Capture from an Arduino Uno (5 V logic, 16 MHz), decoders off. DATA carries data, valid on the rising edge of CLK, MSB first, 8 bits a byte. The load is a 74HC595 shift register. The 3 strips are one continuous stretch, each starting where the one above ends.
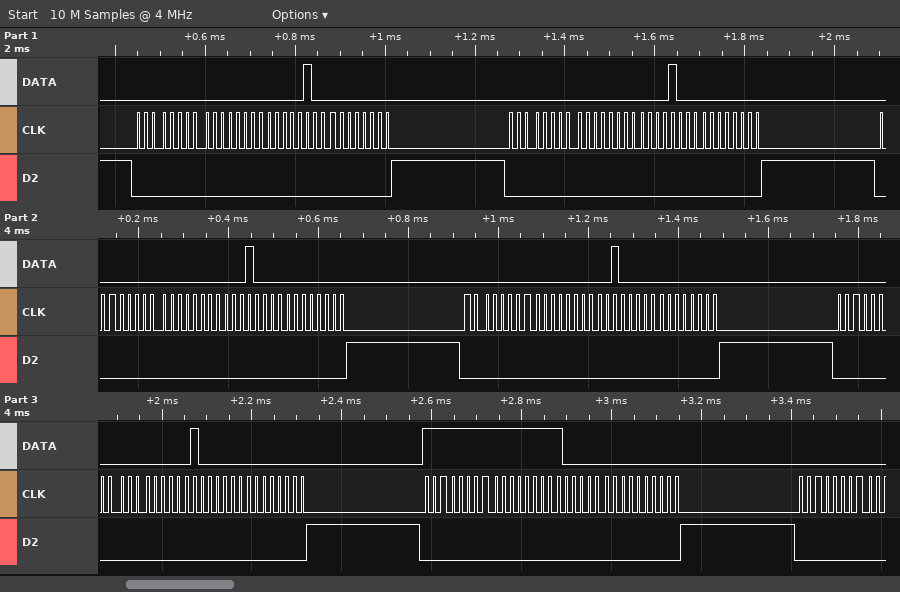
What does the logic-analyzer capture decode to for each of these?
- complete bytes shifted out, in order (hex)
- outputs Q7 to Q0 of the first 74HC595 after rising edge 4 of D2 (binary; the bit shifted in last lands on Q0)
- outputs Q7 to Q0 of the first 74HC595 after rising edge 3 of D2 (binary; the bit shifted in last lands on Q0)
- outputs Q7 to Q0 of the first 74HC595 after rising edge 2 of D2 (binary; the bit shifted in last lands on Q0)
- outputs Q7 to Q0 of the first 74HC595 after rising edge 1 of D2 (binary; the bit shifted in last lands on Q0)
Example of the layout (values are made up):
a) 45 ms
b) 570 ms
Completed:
a) 00 00 04 00 00 00 08 00 00 00 10 00 00 00 20 00 00 00 40 00 FF FF 80 00 00
b) 00000000
c) 00000000
d) 00000000
e) 00000000
